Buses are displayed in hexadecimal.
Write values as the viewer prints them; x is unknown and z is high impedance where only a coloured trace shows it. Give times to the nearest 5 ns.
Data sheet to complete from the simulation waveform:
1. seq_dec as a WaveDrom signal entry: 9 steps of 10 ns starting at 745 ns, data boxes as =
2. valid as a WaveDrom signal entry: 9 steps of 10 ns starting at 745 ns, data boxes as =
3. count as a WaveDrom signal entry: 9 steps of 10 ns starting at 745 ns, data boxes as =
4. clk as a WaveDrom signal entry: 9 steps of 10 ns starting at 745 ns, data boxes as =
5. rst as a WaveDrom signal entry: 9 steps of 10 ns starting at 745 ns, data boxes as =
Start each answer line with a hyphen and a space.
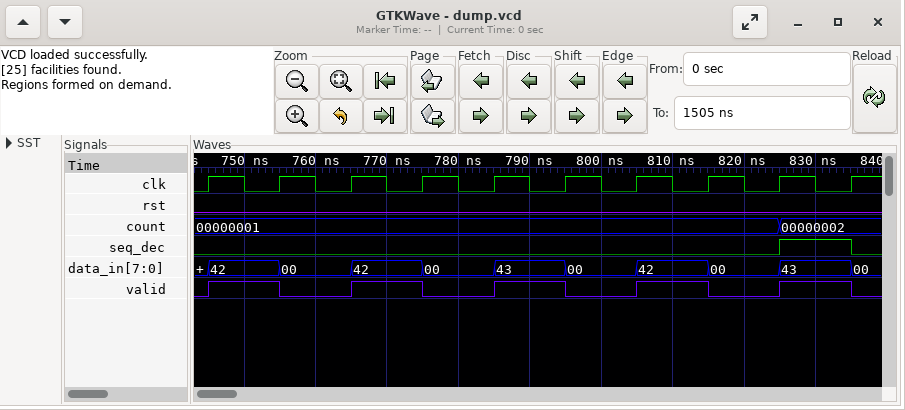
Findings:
- {name: 'seq_dec', wave: '0.......1'}
- {name: 'valid', wave: '101010101'}
- {name: 'count', wave: '=.......=', data: '00000001 00000002'}
- {name: 'clk', wave: 'p........'}
- {name: 'rst', wave: '0........'}
